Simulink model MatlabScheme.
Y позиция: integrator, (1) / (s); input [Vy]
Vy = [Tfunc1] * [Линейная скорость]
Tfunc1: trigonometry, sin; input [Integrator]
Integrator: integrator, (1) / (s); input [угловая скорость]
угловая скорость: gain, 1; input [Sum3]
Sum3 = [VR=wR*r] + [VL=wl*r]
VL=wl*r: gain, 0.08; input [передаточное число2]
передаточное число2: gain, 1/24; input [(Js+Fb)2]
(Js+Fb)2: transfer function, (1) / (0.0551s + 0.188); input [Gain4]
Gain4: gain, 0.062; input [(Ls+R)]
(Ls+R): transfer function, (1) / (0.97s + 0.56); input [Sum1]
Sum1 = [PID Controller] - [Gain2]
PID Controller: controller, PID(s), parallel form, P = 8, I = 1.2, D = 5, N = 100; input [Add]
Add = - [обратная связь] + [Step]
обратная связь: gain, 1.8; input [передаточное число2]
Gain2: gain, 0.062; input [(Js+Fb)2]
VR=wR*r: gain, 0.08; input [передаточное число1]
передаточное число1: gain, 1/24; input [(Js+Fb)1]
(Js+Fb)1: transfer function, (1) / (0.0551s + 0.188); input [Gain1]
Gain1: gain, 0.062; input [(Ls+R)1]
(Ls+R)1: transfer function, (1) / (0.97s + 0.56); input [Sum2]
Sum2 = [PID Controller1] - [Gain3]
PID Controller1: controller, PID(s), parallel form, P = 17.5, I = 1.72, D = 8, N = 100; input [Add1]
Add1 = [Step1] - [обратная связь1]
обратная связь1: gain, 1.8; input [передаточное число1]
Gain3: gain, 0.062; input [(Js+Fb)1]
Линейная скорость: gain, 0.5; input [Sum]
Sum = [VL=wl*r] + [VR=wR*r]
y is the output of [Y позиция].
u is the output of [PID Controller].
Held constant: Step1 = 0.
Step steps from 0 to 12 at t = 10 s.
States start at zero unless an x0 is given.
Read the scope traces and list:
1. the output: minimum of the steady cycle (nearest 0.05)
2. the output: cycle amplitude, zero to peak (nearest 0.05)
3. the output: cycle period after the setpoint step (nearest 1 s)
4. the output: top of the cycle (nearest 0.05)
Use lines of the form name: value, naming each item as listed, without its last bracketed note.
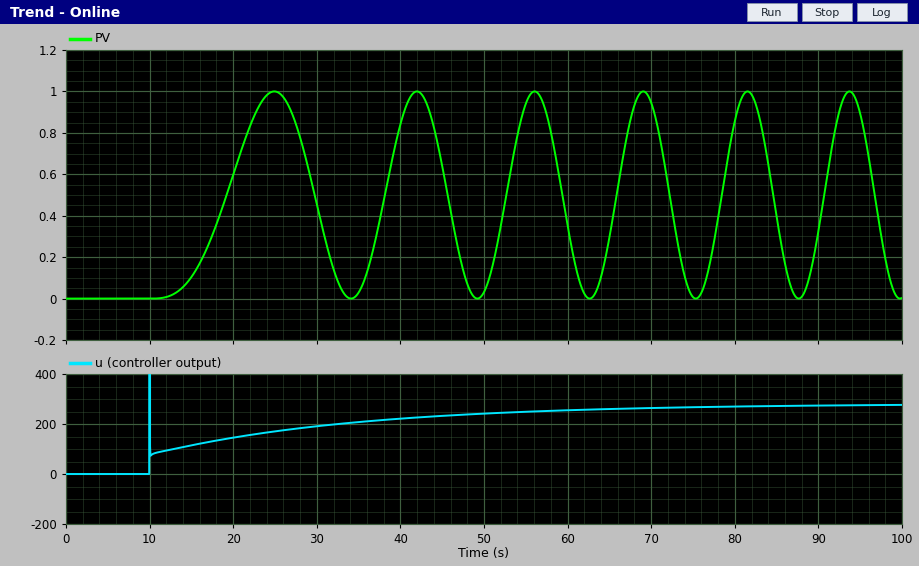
the output: minimum of the steady cycle: 0.00
the output: cycle amplitude, zero to peak: 0.50
the output: cycle period after the setpoint step: 13 s
the output: top of the cycle: 1.00
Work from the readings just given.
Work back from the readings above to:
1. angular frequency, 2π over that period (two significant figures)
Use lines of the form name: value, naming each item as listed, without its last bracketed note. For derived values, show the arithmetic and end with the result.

angular frequency, 2π over that period: 2π / 13 = 0.48 rad/s
